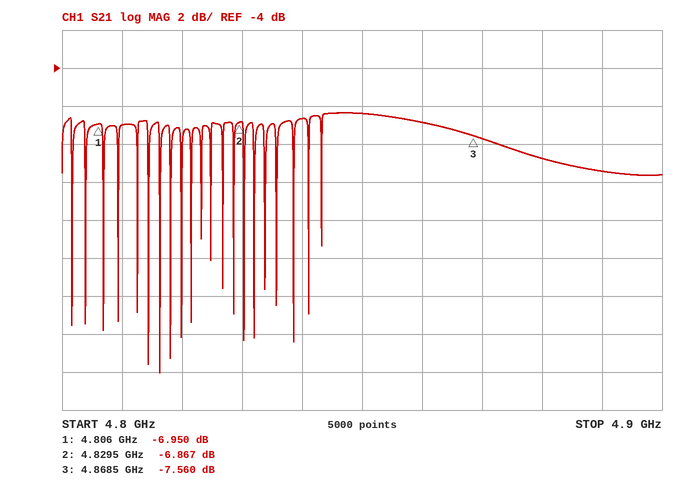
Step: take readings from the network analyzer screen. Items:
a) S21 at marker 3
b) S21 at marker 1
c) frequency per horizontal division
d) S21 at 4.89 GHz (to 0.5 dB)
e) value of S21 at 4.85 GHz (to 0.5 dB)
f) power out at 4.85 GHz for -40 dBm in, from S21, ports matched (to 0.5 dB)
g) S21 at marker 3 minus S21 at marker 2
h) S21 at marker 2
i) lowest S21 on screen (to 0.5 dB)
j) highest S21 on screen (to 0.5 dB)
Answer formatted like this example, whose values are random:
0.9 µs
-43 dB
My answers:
-7.560 dB
-6.950 dB
10 MHz
-9.5 dB
-6.5 dB
-46.5 dBm
-0.693 dB
-6.867 dB
-20.0 dB
-6.5 dB
